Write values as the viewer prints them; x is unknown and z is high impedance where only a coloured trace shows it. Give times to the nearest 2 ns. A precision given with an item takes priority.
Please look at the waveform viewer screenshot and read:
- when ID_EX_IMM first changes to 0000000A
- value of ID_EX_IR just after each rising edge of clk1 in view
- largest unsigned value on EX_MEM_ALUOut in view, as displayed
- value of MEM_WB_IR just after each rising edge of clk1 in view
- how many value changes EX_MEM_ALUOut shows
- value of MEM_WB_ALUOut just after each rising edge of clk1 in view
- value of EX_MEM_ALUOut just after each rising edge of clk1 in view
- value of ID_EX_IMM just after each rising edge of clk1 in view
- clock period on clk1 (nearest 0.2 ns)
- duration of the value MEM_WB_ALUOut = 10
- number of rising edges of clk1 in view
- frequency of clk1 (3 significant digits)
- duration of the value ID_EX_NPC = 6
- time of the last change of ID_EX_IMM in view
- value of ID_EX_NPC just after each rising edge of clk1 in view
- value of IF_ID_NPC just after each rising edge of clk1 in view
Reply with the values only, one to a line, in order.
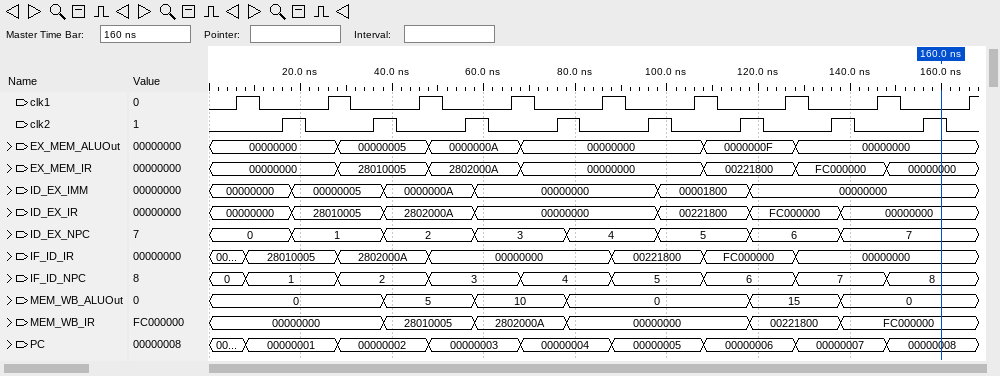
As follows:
38 ns
00000000, 28010005, 2802000A, 00000000, 00000000, 00221800, FC000000, 00000000, 00000000
0000000F
00000000, 00000000, 28010005, 2802000A, 00000000, 00000000, 00221800, FC000000, FC000000
5
0, 0, 5, 10, 0, 0, 15, 0, 0
00000000, 00000000, 00000005, 0000000A, 00000000, 00000000, 0000000F, 00000000, 00000000
00000000, 00000005, 0000000A, 00000000, 00000000, 00001800, 00000000, 00000000, 00000000
20 ns
20 ns
9
50.0 MHz
20 ns
118 ns
0, 1, 2, 3, 4, 5, 6, 7, 7
0, 1, 2, 3, 4, 5, 6, 7, 8
